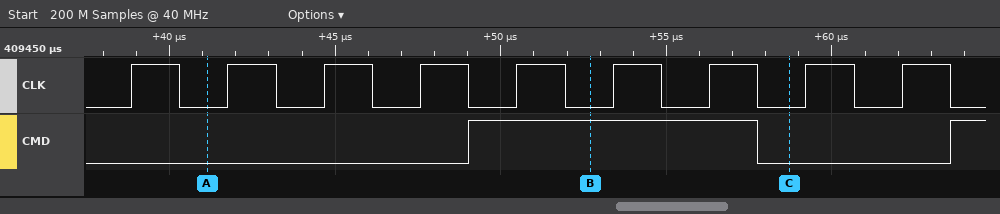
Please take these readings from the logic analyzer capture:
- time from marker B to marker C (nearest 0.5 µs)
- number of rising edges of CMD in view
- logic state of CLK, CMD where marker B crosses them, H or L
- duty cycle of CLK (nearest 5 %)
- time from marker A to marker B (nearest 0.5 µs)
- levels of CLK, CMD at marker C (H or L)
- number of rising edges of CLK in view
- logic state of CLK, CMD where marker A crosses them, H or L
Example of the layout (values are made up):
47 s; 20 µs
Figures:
6 µs; 2; CLK=L, CMD=H; 50 %; 11.5 µs; CLK=L, CMD=L; 9; CLK=L, CMD=L
